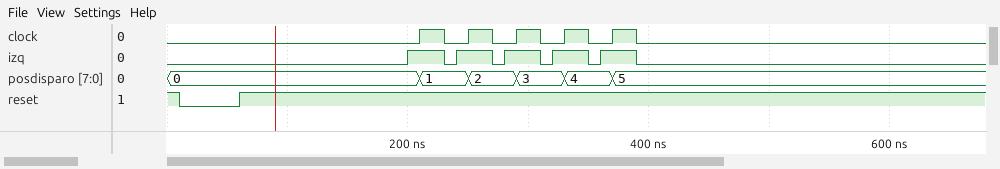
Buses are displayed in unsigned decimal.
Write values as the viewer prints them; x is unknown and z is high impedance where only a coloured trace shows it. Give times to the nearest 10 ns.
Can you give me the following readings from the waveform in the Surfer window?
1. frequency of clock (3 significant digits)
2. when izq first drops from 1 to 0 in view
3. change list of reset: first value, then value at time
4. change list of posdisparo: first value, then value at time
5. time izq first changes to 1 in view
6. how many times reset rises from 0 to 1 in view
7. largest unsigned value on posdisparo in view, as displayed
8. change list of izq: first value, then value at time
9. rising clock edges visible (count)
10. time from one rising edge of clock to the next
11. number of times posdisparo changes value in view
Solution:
25.0 MHz
230 ns
1, 0 at 10 ns, 1 at 60 ns
0, 1 at 210 ns, 2 at 250 ns, 3 at 290 ns, 4 at 330 ns, 5 at 370 ns
200 ns
1
5
0, 1 at 200 ns, 0 at 230 ns, 1 at 240 ns, 0 at 270 ns, 1 at 280 ns, 0 at 310 ns, 1 at 320 ns, 0 at 350 ns, 1 at 360 ns, 0 at 390 ns
5
40 ns
5
